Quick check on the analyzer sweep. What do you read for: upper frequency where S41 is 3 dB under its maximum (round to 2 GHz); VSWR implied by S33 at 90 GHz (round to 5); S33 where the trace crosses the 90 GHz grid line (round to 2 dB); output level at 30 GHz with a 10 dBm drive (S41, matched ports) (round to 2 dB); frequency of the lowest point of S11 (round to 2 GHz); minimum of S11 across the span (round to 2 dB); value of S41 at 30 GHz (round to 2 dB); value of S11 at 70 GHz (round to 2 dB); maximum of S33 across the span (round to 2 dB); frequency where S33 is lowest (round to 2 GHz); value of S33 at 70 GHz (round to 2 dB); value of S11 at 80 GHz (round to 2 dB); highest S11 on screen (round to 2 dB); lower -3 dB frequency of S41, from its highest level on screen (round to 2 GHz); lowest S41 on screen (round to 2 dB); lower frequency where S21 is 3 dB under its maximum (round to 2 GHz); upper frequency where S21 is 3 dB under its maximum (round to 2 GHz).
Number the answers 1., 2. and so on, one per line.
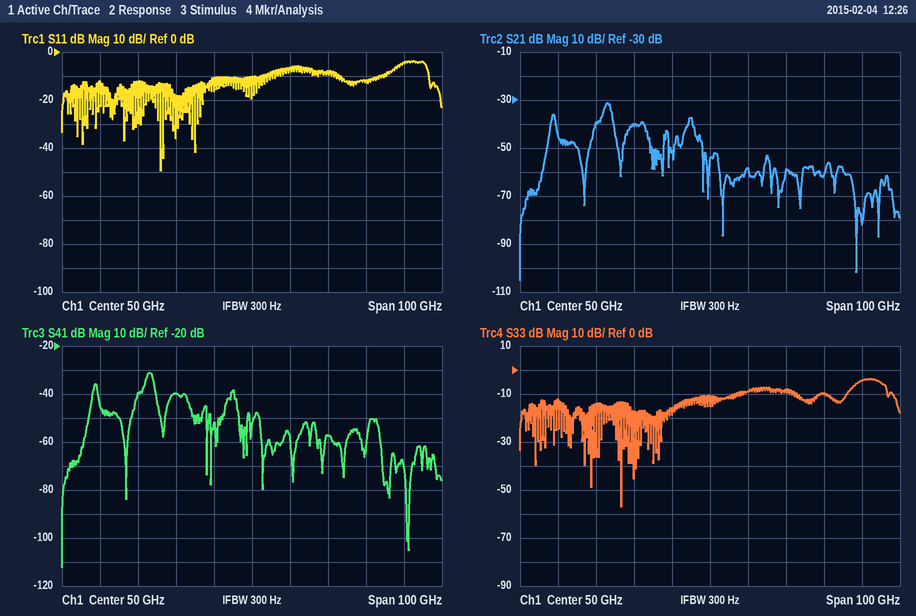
1. 24 GHz
2. 5
3. -4 dB
4. -30 dBm
5. 26 GHz
6. -50 dB
7. -40 dB
8. -8 dB
9. -4 dB
10. 26 GHz
11. -8 dB
12. -12 dB
13. -4 dB
14. 22 GHz
15. -112 dB
16. 22 GHz
17. 24 GHz
